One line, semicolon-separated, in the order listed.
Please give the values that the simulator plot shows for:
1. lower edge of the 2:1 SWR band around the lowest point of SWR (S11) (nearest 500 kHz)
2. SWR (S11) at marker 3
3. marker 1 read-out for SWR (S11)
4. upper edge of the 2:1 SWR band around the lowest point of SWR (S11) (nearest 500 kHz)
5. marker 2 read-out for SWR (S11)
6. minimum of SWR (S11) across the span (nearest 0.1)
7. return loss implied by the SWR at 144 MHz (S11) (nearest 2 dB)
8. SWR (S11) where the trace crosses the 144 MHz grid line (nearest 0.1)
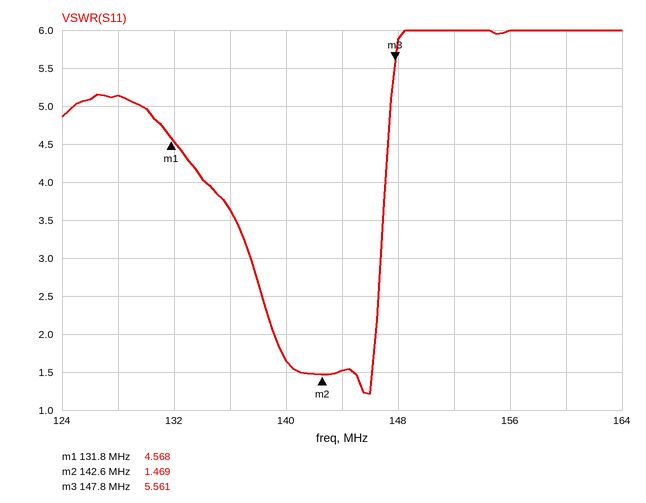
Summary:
139.0 MHz; 5.561; 4.568; 146.5 MHz; 1.469; 1.2; 14 dB; 1.5
